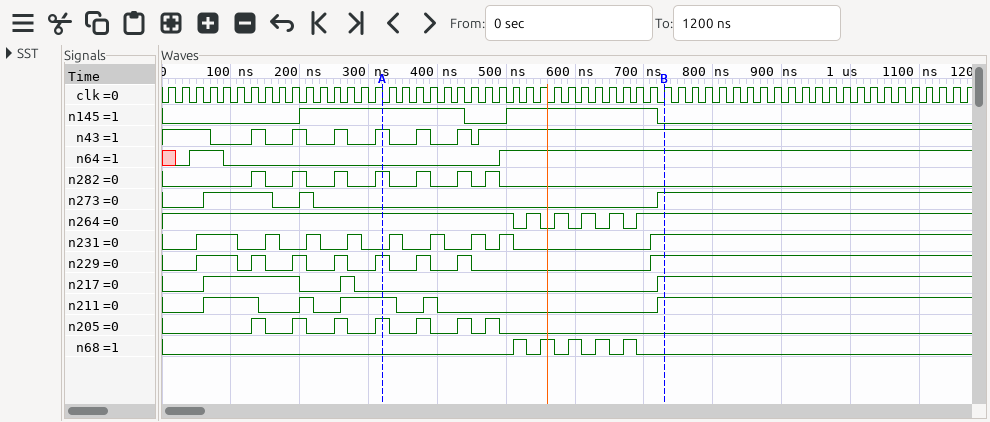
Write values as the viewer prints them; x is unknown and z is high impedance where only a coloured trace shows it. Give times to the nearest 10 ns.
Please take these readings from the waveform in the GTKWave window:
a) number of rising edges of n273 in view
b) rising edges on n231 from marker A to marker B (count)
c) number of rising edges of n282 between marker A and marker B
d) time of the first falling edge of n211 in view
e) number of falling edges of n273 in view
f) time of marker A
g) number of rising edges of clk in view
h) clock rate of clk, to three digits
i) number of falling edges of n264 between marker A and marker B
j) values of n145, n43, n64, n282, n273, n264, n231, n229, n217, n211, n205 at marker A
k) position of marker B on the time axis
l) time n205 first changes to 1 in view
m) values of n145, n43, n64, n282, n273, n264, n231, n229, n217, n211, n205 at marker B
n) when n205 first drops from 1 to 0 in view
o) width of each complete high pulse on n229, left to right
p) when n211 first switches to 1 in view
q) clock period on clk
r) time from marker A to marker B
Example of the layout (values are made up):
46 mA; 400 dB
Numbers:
3; 5; 3; 140 ns; 2; 320 ns; 59; 50.0 MHz; 5; n145=1, n43=1, n64=0, n282=1, n273=0, n264=1, n231=0, n229=1, n217=0, n211=1, n205=1; 730 ns; 130 ns; n145=0, n43=1, n64=1, n282=0, n273=1, n264=1, n231=1, n229=1, n217=1, n211=1, n205=0; 150 ns; 60 ns, 20 ns, 20 ns, 20 ns, 20 ns, 20 ns, 20 ns; 60 ns; 20 ns; 410 ns
